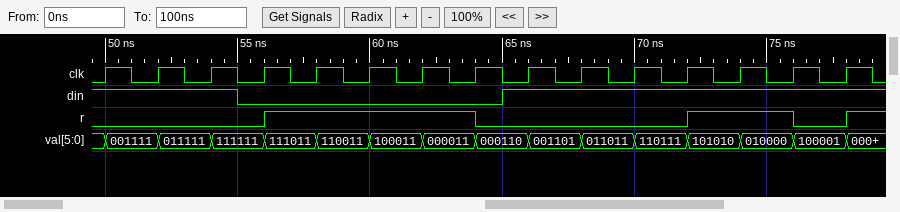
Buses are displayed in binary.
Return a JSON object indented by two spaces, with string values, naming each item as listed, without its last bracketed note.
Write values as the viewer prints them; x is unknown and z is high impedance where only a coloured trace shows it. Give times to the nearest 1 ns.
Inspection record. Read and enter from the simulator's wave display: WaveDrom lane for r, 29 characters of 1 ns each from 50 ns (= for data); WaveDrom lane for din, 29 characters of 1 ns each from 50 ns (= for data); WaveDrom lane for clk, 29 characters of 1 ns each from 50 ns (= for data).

{
  "WaveDrom lane for r, 29 characters of 1 ns each from 50 ns": "{name: 'r', wave: '0.....1.......0.......1...0.1'}",
  "WaveDrom lane for din, 29 characters of 1 ns each from 50 ns": "{name: 'din', wave: '1....0.........1.............'}",
  "WaveDrom lane for clk, 29 characters of 1 ns each from 50 ns": "{name: 'clk', wave: '10101010101010101010101010101'}"
}
